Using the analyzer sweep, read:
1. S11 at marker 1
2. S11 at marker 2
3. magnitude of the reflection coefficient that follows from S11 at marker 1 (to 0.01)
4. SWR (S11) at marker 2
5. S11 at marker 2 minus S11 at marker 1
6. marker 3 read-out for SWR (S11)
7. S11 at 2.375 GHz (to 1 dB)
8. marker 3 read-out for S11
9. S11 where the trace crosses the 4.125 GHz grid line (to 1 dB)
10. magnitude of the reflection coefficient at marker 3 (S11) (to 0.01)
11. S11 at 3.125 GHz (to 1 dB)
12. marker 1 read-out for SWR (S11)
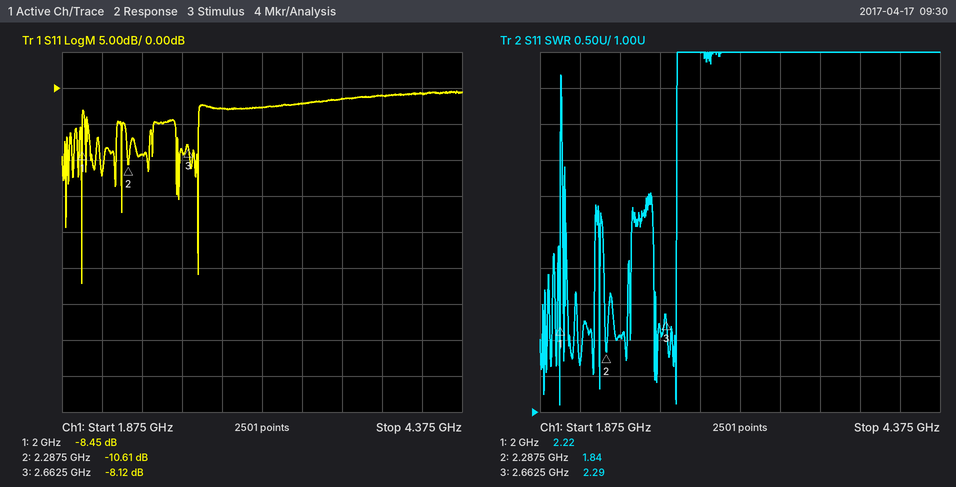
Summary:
-8.45 dB
-10.61 dB
0.38
1.84
-2.16 dB
2.29
-9 dB
-8.12 dB
-1 dB
0.39
-3 dB
2.22
